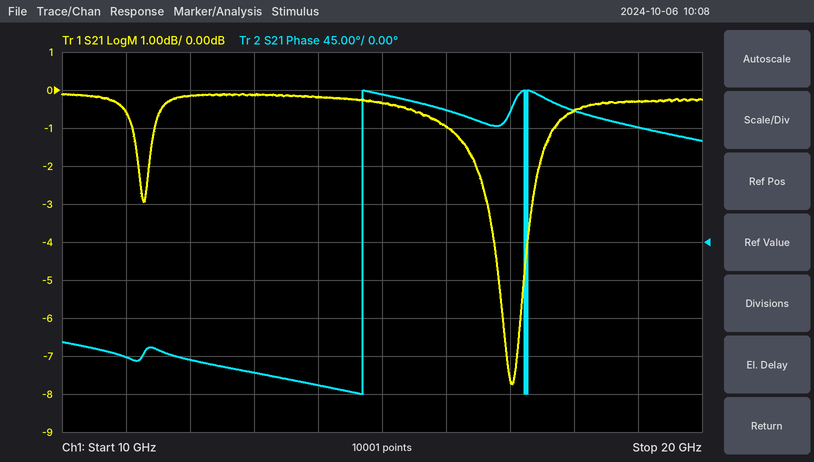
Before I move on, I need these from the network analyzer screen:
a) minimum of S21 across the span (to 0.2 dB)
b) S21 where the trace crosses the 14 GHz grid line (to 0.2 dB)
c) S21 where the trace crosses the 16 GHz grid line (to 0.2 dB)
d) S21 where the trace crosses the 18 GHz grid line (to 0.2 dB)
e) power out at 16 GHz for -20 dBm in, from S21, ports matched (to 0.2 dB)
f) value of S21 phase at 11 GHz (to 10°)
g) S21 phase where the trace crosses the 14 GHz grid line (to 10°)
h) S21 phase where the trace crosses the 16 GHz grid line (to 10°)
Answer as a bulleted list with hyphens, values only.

- -7.8 dB
- -0.2 dB
- -1.0 dB
- -0.6 dB
- -21.0 dBm
- -140°
- -170°
- 160°
